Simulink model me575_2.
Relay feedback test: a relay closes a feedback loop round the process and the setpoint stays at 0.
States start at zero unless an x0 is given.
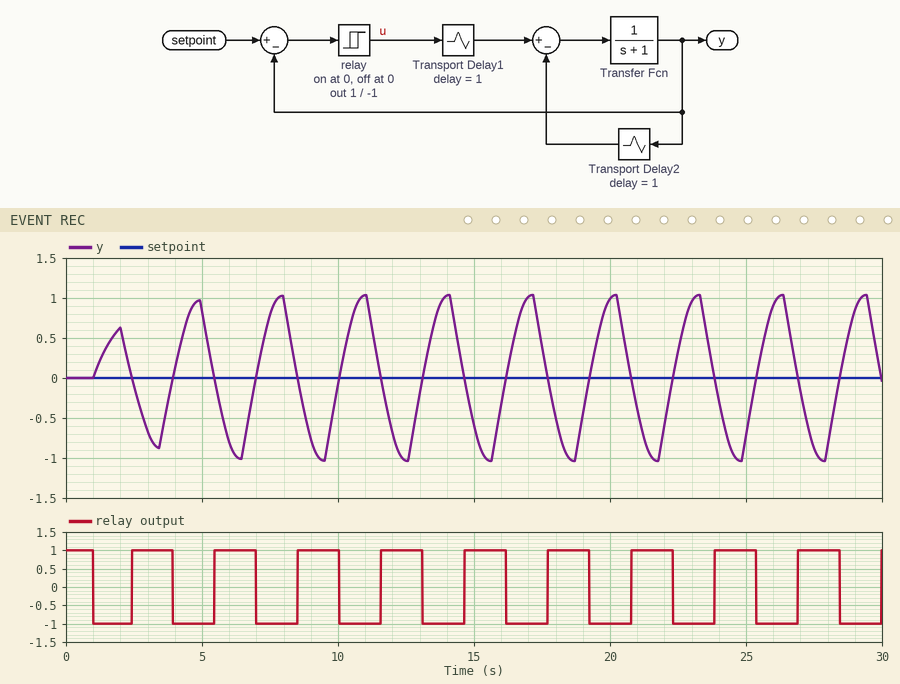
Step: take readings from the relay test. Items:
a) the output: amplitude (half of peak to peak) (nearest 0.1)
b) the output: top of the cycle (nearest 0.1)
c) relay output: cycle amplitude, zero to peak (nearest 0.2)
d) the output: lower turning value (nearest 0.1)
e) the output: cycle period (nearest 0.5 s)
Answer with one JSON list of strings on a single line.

["1.0", "1.0", "1.0", "-1.0", "3.0 s"]
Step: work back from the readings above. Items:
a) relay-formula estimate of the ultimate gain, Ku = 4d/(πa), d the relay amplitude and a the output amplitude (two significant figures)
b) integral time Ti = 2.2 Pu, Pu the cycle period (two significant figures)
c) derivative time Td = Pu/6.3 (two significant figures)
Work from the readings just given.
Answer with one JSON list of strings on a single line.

["1.3", "6.6 s", "0.48 s"]
